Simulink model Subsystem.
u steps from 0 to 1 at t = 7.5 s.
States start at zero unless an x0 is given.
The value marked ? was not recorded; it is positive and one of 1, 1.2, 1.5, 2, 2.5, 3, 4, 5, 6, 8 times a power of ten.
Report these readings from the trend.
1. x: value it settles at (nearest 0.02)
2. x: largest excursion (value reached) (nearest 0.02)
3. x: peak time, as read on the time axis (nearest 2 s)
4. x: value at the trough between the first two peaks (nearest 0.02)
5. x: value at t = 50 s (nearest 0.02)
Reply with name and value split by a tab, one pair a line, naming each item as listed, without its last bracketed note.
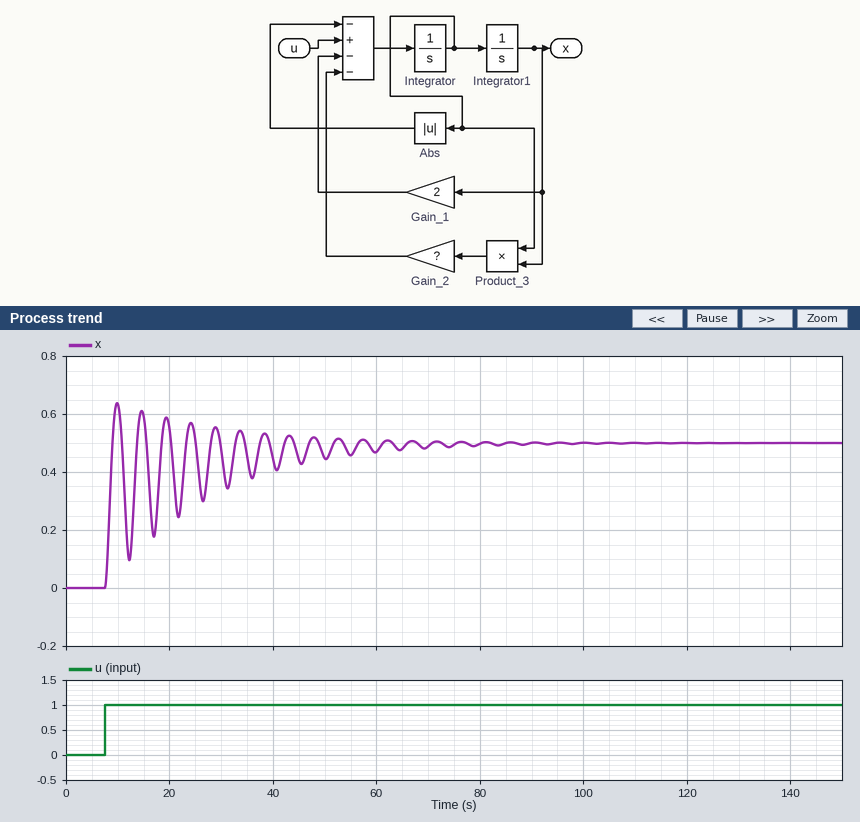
x: value it settles at	0.50
x: largest excursion (value reached)	0.64
x: peak time, as read on the time axis	10 s
x: value at the trough between the first two peaks	0.10
x: value at t = 50 s	0.44
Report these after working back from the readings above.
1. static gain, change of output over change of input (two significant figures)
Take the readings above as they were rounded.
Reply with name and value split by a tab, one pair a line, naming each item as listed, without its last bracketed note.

static gain, change of output over change of input	0.50
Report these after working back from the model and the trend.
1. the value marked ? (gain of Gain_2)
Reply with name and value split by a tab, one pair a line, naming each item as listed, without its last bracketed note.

the value marked ?	0.2
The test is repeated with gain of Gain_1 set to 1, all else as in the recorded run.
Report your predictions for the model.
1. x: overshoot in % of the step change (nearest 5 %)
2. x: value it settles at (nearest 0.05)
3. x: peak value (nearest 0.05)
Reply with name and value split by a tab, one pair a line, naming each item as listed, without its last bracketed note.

x: overshoot in % of the step change	10 %
x: value it settles at	1.00
x: peak value	1.10
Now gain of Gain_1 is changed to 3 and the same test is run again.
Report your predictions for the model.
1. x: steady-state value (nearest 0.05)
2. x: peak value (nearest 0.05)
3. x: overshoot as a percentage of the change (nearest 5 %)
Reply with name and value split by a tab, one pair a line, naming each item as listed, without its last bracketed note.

x: steady-state value	0.35
x: peak value	0.45
x: overshoot as a percentage of the change	35 %
